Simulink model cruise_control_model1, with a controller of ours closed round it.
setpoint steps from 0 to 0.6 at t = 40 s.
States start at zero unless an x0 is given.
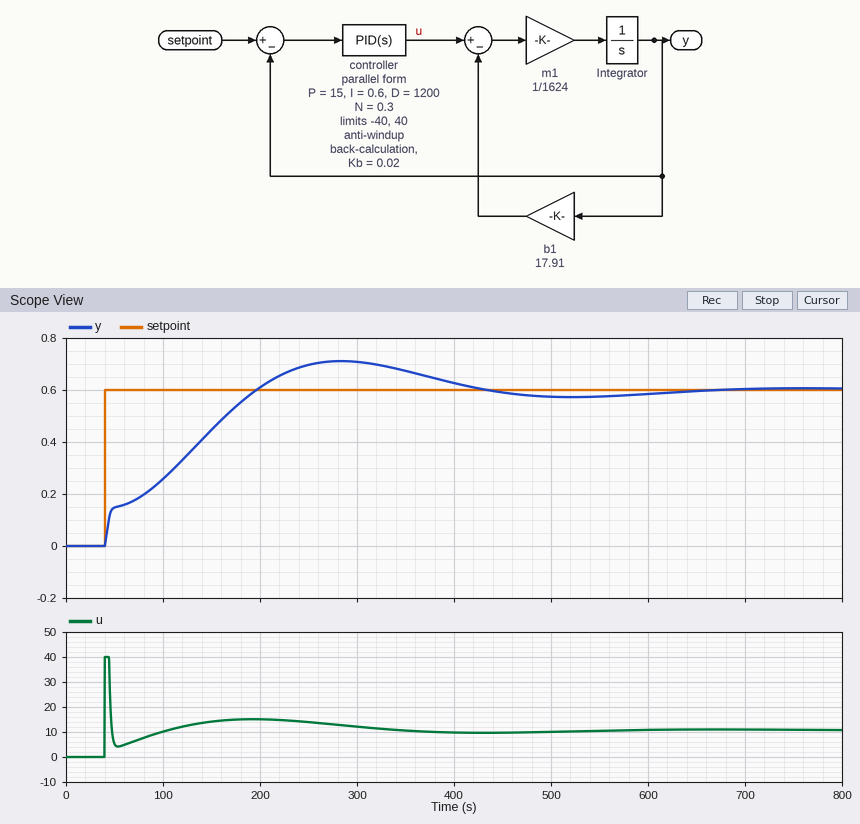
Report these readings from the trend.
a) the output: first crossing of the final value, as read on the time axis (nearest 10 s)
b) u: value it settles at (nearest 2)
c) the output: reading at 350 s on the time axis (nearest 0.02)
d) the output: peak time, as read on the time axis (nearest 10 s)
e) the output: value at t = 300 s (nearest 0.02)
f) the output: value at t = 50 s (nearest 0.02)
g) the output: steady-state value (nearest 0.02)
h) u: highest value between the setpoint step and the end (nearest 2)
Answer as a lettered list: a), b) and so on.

a) 200 s
b) 10
c) 0.68
d) 280 s
e) 0.70
f) 0.14
g) 0.60
h) 40
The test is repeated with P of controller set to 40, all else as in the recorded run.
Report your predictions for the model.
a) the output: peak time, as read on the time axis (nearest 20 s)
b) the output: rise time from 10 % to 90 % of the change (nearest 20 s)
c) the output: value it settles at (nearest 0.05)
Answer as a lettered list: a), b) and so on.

a) 300 s
b) 140 s
c) 0.60
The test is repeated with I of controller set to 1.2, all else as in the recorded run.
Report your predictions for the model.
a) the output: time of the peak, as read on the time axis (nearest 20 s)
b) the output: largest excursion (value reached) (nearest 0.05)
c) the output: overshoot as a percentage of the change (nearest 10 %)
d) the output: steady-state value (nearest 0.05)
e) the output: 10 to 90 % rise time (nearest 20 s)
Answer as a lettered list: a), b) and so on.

a) 200 s
b) 0.75
c) 30 %
d) 0.60
e) 80 s
